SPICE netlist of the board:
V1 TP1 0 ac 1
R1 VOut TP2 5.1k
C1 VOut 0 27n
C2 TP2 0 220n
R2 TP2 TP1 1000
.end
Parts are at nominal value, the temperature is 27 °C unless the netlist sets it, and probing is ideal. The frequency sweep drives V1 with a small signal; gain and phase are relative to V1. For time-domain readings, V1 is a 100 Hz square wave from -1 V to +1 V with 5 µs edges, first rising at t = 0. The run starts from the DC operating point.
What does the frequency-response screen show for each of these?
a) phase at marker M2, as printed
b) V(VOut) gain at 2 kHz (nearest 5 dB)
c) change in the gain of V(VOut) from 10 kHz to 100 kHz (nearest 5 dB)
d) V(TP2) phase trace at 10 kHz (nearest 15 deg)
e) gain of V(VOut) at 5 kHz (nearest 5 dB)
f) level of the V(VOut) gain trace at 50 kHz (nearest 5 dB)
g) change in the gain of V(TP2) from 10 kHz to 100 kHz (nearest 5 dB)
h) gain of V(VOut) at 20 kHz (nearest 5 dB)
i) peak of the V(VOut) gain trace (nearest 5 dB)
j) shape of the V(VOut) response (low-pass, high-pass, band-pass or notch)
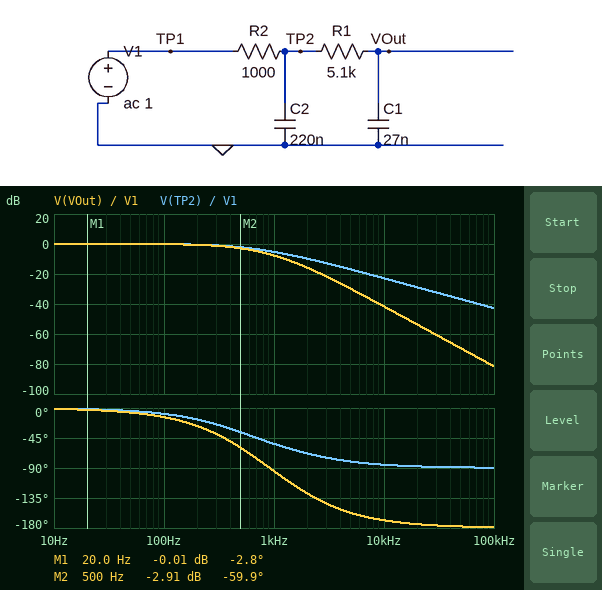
-59.9 deg
-15 dB
-40 dB
-90 deg
-30 dB
-70 dB
-20 dB
-55 dB
0 dB
low-pass
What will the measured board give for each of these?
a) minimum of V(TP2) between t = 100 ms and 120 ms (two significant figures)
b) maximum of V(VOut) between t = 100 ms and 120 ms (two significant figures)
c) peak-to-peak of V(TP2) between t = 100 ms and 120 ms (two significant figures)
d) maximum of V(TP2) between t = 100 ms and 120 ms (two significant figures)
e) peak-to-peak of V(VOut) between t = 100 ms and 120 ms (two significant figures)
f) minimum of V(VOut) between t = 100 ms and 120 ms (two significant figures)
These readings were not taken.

-1.0 V
1.0 V
2.0 V
1.0 V
2.0 V
-1.0 V
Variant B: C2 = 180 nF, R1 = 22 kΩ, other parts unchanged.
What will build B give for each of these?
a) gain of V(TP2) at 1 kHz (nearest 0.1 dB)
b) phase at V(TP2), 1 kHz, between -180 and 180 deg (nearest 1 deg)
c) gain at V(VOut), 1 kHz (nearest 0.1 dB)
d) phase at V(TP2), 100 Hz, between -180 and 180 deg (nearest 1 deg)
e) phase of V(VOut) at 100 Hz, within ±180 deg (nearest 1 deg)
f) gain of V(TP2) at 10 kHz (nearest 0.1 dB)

-3.8 dB
-48 deg
-15.5 dB
-7 deg
-28 deg
-21.1 dB
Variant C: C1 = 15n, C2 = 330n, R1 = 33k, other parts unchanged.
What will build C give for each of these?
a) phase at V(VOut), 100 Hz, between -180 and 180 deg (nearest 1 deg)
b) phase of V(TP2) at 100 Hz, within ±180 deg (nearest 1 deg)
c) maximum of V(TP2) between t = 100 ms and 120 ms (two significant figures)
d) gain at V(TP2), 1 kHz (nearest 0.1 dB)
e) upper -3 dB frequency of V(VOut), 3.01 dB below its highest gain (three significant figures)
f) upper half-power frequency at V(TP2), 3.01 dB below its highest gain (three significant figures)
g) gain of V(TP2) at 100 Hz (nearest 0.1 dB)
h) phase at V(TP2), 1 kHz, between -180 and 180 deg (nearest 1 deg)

-29 deg
-12 deg
1.0 V
-7.3 dB
240 Hz
465 Hz
-0.2 dB
-64 deg
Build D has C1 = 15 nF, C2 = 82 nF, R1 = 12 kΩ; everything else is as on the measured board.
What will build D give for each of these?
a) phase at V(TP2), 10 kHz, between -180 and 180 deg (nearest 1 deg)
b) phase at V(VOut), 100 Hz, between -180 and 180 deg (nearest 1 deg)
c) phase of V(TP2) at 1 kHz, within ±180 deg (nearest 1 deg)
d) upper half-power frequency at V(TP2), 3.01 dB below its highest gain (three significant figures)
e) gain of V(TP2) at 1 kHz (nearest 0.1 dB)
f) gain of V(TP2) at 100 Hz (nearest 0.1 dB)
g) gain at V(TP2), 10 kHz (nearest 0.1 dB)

-78 deg
-10 deg
-28 deg
1.74 kHz
-1.5 dB
0 dB
-14.4 dB
